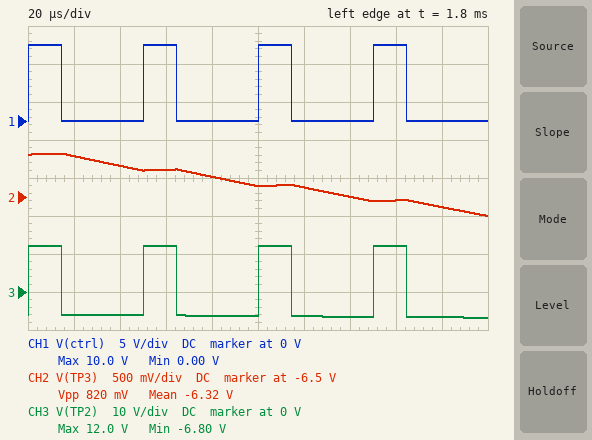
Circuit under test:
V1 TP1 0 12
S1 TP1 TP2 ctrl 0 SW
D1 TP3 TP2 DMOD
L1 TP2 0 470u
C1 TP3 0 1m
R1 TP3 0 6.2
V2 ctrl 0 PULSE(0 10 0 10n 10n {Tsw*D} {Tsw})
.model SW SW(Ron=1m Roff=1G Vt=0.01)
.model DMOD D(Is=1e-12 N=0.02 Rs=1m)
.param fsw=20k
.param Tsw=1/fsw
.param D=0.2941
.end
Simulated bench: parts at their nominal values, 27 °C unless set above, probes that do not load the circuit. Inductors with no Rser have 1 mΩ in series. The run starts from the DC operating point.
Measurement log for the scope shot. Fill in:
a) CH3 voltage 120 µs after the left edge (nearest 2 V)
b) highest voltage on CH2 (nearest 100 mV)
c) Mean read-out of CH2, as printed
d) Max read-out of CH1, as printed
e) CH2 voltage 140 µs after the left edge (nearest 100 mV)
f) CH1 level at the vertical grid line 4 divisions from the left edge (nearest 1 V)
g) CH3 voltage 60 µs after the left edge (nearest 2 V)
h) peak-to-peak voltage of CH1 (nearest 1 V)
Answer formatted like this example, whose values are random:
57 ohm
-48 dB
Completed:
-6 V
-5.9 V
-6.32 V
10.0 V
-6.5 V
0 V
12 V
10 V
